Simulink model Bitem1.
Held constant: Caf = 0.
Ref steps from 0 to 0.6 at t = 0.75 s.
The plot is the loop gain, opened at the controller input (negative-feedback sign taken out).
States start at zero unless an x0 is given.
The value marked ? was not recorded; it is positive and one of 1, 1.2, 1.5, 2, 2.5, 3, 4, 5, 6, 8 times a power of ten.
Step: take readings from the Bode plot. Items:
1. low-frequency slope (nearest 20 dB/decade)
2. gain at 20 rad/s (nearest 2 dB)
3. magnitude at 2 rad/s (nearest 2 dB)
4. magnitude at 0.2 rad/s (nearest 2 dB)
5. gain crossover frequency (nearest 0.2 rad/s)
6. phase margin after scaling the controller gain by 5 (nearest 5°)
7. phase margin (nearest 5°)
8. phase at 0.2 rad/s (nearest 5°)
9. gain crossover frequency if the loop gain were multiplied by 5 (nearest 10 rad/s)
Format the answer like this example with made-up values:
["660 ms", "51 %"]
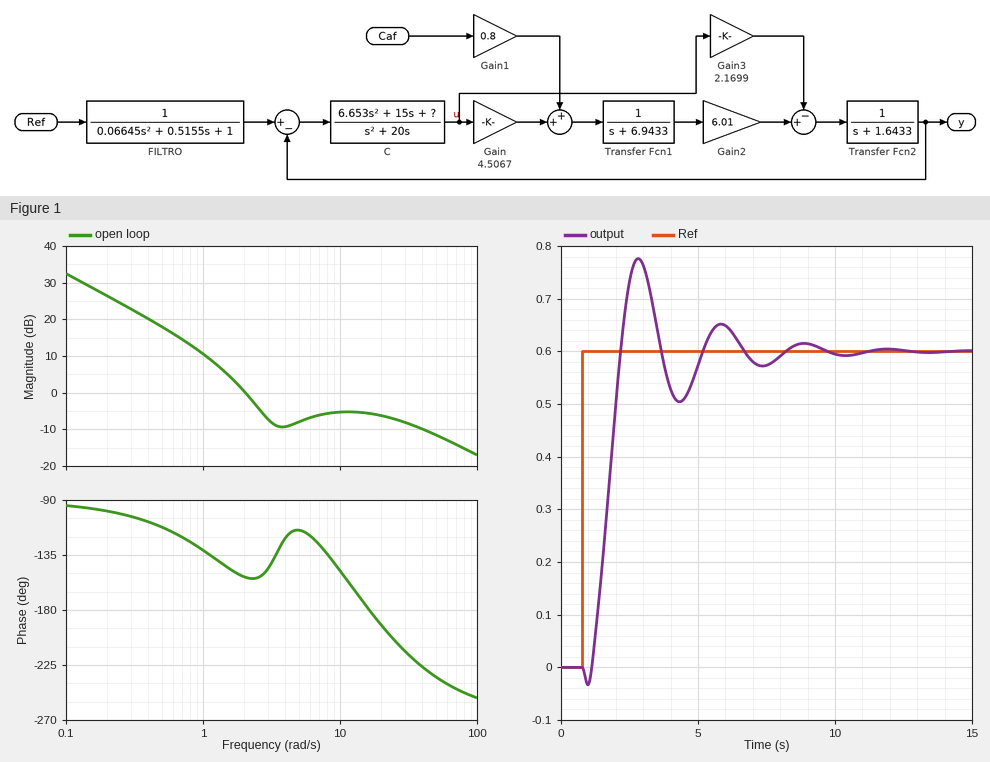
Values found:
["-20 dB/decade", "-6 dB", "0 dB", "26 dB", "2.0 rad/s", "-65°", "25°", "-100°", "70 rad/s"]
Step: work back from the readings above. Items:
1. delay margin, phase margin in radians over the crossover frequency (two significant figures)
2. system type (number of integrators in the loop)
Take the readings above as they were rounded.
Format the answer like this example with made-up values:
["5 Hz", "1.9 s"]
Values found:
["0.22 s", "1"]
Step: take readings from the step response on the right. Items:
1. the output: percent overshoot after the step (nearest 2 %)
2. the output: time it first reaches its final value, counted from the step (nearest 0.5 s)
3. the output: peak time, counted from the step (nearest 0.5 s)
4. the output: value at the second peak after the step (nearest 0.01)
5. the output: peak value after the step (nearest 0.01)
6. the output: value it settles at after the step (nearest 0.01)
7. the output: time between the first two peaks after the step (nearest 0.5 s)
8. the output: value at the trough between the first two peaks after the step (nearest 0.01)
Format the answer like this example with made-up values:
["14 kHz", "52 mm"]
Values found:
["30 %", "1.5 s", "2.0 s", "0.65", "0.78", "0.60", "3.0 s", "0.50"]
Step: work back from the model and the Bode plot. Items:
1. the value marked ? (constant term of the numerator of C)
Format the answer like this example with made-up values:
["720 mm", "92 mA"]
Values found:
["80"]
